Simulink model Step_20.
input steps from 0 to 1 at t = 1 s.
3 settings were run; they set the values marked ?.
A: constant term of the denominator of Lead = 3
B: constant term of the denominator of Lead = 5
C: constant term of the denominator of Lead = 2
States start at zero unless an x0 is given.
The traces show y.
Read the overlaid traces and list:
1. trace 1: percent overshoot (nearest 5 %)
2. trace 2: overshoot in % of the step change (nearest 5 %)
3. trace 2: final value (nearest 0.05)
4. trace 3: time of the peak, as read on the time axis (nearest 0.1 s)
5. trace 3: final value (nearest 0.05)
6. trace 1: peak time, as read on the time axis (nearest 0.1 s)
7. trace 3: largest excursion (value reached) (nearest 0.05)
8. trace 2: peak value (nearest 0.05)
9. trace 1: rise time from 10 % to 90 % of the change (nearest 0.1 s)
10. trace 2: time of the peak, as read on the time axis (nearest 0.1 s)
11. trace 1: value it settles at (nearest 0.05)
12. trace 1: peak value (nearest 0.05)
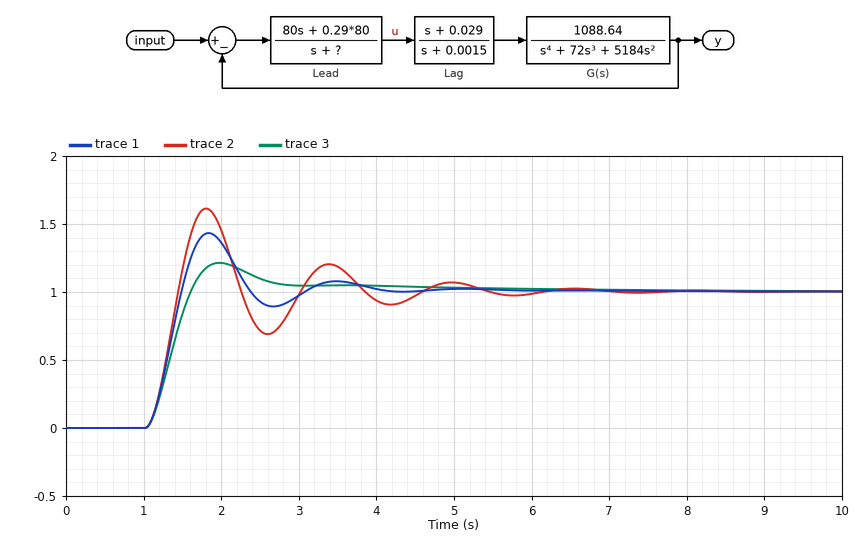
45 %
60 %
1.00
2.0 s
1.00
1.8 s
1.20
1.60
0.3 s
1.8 s
1.00
1.45
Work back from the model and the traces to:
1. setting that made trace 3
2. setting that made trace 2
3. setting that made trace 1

B
C
A
